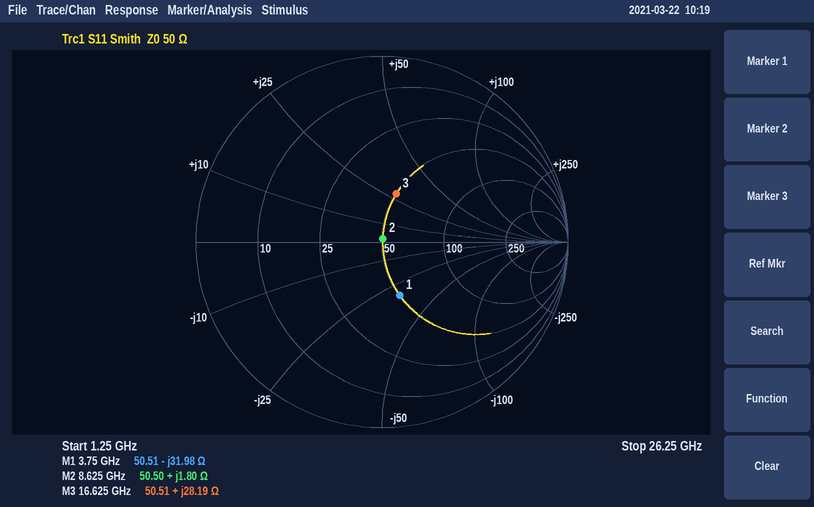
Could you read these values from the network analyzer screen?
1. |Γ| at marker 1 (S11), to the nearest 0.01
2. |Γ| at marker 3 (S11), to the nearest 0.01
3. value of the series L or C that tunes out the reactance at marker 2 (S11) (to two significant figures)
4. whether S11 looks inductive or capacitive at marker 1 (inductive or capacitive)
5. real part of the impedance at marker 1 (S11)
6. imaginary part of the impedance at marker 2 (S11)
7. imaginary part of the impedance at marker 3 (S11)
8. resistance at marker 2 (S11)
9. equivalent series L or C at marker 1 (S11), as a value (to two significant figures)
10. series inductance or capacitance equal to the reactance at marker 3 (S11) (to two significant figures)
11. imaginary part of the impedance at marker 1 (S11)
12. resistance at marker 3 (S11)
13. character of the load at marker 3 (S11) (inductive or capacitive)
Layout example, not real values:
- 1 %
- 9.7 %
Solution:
- 0.30
- 0.27
- 10 pF
- capacitive
- 50.51 Ω
- +1.80 Ω
- +28.19 Ω
- 50.50 Ω
- 1.3 pF
- 270 pH
- -31.98 Ω
- 50.51 Ω
- inductive
